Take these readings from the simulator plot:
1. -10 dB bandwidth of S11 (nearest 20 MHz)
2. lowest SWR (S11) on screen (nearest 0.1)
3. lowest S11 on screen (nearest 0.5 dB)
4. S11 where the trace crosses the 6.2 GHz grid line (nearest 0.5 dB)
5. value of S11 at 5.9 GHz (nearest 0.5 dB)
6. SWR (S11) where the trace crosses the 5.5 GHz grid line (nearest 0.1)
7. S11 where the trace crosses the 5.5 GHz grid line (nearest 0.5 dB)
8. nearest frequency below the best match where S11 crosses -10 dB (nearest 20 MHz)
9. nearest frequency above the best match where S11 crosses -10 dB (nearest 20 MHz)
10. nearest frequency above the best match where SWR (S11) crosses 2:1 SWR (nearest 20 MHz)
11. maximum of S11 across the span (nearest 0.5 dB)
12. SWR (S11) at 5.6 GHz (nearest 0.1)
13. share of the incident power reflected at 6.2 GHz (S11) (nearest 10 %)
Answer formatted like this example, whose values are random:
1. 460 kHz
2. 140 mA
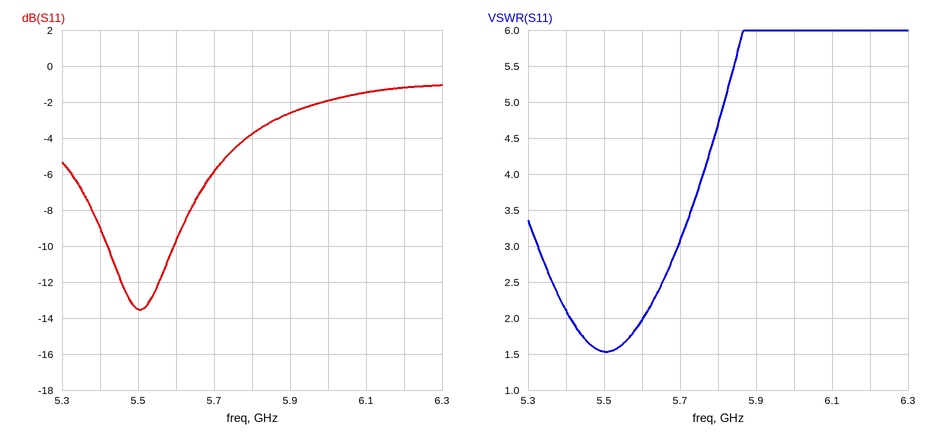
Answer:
1. 180 MHz
2. 1.5
3. -13.5 dB
4. -1.0 dB
5. -2.5 dB
6. 1.5
7. -13.5 dB
8. 5.42 GHz
9. 5.60 GHz
10. 5.60 GHz
11. -1.0 dB
12. 2.0
13. 80 %
